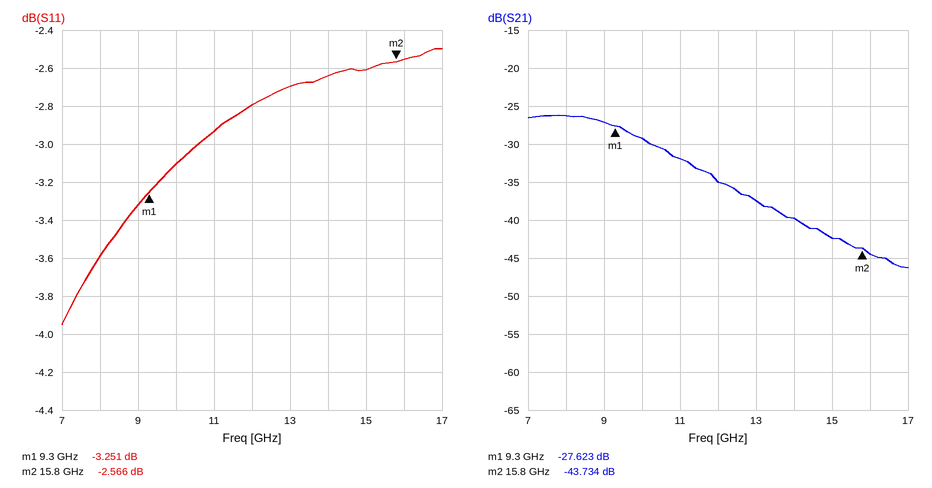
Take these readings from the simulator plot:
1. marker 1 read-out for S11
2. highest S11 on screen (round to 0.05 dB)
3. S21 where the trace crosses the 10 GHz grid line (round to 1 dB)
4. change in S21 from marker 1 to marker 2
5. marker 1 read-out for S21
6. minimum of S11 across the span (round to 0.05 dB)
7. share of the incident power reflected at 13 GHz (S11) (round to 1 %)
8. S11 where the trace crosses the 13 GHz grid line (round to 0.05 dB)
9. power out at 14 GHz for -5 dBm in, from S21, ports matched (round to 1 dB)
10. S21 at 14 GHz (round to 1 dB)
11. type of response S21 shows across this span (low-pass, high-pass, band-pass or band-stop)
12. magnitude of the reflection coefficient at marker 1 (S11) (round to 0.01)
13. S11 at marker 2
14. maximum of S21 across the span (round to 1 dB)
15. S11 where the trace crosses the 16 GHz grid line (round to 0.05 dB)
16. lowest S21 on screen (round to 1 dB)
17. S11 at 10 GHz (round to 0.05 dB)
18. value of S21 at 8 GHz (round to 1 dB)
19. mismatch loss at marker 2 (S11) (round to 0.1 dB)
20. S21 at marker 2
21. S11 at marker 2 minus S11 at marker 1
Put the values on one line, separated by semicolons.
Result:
-3.251 dB; -2.50 dB; -29 dB; -16.111 dB; -27.623 dB; -3.95 dB; 54 %; -2.70 dB; -45 dBm; -40 dB; low-pass; 0.69; -2.566 dB; -26 dB; -2.55 dB; -46 dB; -3.10 dB; -26 dB; 3.5 dB; -43.734 dB; 0.685 dB
